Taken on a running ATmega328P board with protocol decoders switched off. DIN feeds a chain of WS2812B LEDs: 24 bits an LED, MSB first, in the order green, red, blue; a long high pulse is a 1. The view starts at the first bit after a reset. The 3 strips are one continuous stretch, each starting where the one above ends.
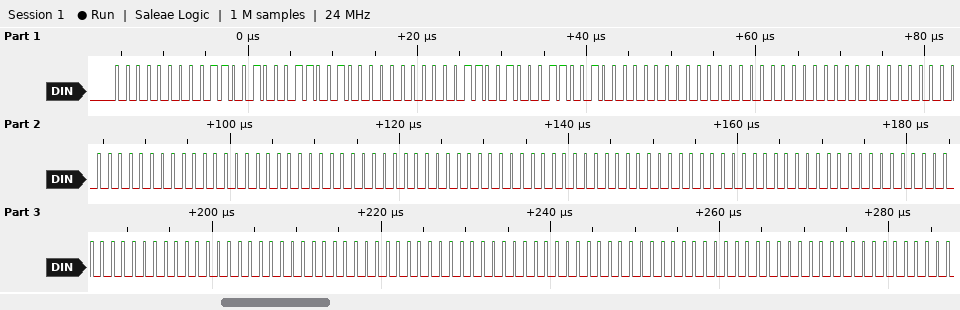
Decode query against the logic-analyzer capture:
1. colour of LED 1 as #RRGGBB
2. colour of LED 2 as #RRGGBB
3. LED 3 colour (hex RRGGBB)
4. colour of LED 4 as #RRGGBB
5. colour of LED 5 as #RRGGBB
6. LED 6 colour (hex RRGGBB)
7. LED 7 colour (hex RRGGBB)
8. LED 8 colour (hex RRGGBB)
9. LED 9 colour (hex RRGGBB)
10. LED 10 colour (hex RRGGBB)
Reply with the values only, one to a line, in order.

#640064
#640064
#000000
#000000
#000000
#000000
#000000
#000000
#000000
#000000
